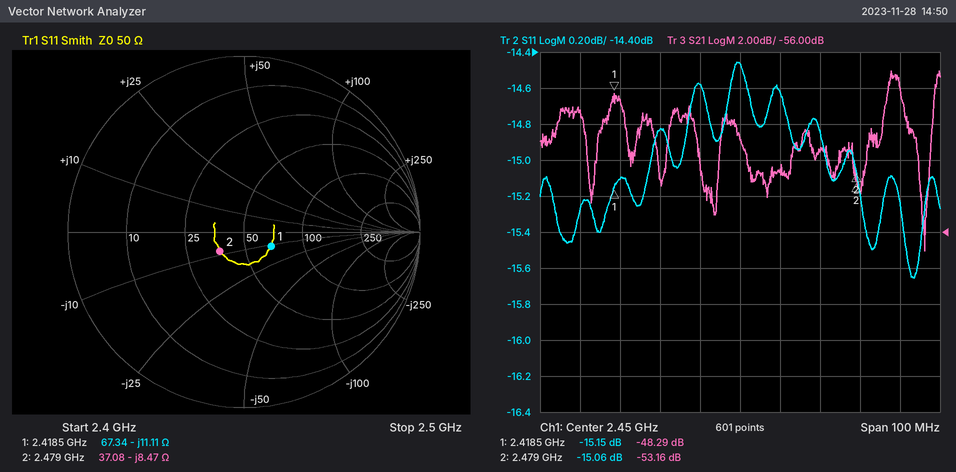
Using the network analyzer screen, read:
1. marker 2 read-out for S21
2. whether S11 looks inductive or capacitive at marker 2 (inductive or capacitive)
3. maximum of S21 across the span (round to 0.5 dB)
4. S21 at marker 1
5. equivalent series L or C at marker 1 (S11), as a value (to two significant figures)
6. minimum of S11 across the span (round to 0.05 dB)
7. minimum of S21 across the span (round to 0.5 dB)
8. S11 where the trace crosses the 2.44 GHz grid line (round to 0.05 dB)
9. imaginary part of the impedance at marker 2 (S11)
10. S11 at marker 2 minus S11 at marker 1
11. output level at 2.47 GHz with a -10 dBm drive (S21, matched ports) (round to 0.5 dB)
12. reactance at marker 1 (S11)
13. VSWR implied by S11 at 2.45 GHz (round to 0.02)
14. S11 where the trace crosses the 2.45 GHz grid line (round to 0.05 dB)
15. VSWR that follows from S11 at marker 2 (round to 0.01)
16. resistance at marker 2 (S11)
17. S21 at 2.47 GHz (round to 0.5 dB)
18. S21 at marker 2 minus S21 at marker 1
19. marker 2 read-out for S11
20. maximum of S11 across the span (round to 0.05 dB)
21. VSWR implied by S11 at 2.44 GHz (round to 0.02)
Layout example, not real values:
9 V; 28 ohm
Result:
-53.16 dB; capacitive; -47.0 dB; -48.29 dB; 5.9 pF; -15.65 dB; -57.0 dB; -14.60 dB; -8.47 Ω; 0.09 dB; -61.5 dBm; -11.11 Ω; 1.46; -14.45 dB; 1.43; 37.08 Ω; -51.5 dB; -4.87 dB; -15.06 dB; -14.45 dB; 1.46
